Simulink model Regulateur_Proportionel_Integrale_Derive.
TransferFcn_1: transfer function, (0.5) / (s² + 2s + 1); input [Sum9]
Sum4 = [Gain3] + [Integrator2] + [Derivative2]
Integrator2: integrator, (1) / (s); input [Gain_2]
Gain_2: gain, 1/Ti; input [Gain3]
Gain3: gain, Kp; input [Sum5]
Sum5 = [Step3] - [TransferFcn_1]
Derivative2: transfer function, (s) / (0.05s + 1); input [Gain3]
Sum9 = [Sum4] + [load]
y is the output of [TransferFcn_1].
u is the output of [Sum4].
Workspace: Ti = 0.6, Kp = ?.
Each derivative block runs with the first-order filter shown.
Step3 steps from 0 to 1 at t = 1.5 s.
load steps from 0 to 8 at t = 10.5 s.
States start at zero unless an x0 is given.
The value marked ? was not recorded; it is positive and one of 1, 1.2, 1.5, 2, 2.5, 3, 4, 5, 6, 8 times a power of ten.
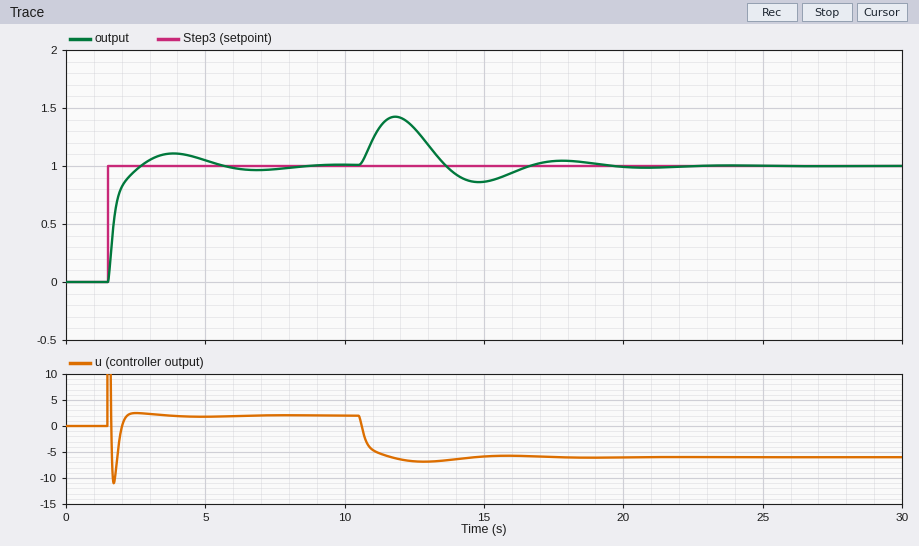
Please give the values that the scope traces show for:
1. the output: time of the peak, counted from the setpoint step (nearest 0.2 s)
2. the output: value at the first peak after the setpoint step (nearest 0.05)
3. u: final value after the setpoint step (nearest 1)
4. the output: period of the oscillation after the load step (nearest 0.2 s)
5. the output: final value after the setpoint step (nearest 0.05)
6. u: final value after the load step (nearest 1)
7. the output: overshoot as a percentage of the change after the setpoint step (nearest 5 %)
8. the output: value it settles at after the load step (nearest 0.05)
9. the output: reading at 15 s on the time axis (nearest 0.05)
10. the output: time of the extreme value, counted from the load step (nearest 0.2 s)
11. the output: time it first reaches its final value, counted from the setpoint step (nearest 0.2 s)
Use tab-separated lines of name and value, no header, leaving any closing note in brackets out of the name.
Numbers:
the output: time of the peak, counted from the setpoint step	2.4 s
the output: value at the first peak after the setpoint step	1.10
u: final value after the setpoint step	2
the output: period of the oscillation after the load step	6.0 s
the output: final value after the setpoint step	1.00
u: final value after the load step	-6
the output: overshoot as a percentage of the change after the setpoint step	10 %
the output: value it settles at after the load step	1.00
the output: reading at 15 s on the time axis	0.85
the output: time of the extreme value, counted from the load step	1.4 s
the output: time it first reaches its final value, counted from the setpoint step	1.2 s
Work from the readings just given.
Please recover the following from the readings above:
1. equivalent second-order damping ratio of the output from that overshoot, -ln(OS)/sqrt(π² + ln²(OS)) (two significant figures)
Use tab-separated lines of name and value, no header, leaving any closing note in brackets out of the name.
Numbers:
equivalent second-order damping ratio of the output from that overshoot, -ln(OS)/sqrt(π² + ln²(OS))	0.59
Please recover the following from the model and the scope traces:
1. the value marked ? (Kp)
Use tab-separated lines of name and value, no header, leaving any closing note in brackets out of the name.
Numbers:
the value marked ?	8
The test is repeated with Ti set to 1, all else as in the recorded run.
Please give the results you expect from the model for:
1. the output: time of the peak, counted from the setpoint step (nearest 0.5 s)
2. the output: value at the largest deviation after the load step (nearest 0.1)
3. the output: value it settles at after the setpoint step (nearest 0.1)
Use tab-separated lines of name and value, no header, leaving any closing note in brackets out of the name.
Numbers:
the output: time of the peak, counted from the setpoint step	3.5 s
the output: value at the largest deviation after the load step	1.5
the output: value it settles at after the setpoint step	1.0
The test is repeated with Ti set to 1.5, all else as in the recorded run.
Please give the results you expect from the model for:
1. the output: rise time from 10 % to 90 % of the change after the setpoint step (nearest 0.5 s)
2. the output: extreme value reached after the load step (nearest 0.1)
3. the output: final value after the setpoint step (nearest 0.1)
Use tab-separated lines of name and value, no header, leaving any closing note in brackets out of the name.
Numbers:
the output: rise time from 10 % to 90 % of the change after the setpoint step	1.5 s
the output: extreme value reached after the load step	1.5
the output: final value after the setpoint step	1.0
